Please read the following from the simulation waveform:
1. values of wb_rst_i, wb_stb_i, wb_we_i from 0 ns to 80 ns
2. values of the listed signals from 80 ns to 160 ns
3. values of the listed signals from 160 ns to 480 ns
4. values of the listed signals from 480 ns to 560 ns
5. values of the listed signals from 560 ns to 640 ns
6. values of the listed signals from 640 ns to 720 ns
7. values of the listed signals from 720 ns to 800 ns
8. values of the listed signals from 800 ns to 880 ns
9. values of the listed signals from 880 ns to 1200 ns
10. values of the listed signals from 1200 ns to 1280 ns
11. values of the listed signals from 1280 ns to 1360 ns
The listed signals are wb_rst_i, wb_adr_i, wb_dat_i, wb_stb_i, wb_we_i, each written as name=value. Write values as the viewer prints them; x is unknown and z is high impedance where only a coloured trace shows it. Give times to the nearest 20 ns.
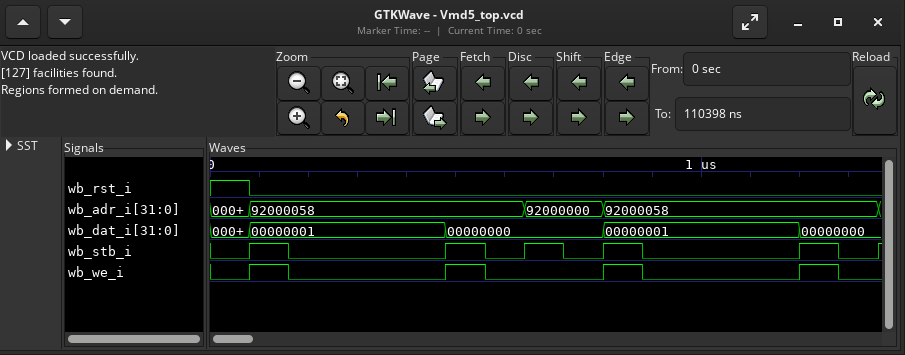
wb_rst_i=1, wb_stb_i=0, wb_we_i=0
wb_rst_i=0, wb_adr_i=92000058, wb_dat_i=00000001, wb_stb_i=1, wb_we_i=1
wb_rst_i=0, wb_adr_i=92000058, wb_dat_i=00000001, wb_stb_i=0, wb_we_i=0
wb_rst_i=0, wb_adr_i=92000058, wb_dat_i=00000000, wb_stb_i=1, wb_we_i=1
wb_rst_i=0, wb_adr_i=92000058, wb_dat_i=00000000, wb_stb_i=0, wb_we_i=0
wb_rst_i=0, wb_adr_i=92000000, wb_dat_i=00000000, wb_stb_i=1, wb_we_i=0
wb_rst_i=0, wb_adr_i=92000000, wb_dat_i=00000000, wb_stb_i=0, wb_we_i=0
wb_rst_i=0, wb_adr_i=92000058, wb_dat_i=00000001, wb_stb_i=1, wb_we_i=1
wb_rst_i=0, wb_adr_i=92000058, wb_dat_i=00000001, wb_stb_i=0, wb_we_i=0
wb_rst_i=0, wb_adr_i=92000058, wb_dat_i=00000000, wb_stb_i=1, wb_we_i=1
wb_rst_i=0, wb_adr_i=92000058, wb_dat_i=00000000, wb_stb_i=0, wb_we_i=0
